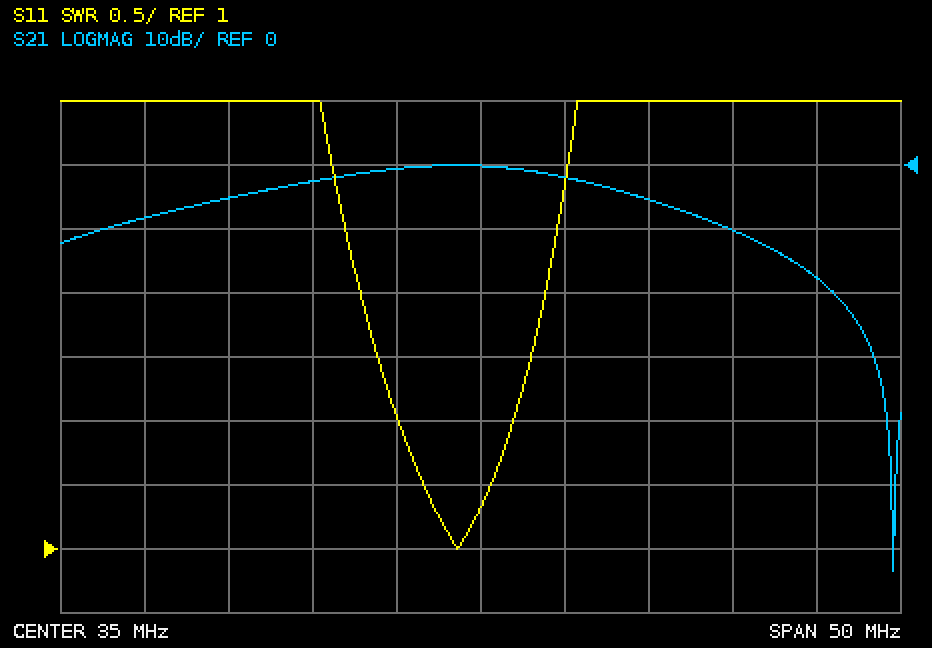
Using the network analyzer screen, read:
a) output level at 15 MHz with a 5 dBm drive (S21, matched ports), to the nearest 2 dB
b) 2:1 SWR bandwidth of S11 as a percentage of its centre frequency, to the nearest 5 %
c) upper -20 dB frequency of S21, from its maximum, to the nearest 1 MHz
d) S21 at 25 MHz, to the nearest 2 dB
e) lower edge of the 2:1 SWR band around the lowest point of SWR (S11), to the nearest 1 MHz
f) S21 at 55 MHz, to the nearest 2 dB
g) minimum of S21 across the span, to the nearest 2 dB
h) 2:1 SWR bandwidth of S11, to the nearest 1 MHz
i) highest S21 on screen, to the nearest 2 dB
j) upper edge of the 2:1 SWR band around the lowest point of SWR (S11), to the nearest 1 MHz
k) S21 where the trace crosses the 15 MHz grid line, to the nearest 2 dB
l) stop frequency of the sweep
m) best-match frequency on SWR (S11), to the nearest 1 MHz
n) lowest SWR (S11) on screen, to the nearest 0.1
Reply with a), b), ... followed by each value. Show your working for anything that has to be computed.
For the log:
a) 5 dBm + (-8 dB) = -4 dBm
b) 7 MHz / 33.5 MHz ≈ 20.9 %, so 20 % to the nearest 5 %
c) 56 MHz
d) -2 dB
e) 30 MHz
f) -18 dB
g) -64 dB
h) 37 MHz − 30 MHz = 7 MHz
i) 0 dB
j) 37 MHz
k) -8 dB
l) 60 MHz
m) 34 MHz
n) 1.0
